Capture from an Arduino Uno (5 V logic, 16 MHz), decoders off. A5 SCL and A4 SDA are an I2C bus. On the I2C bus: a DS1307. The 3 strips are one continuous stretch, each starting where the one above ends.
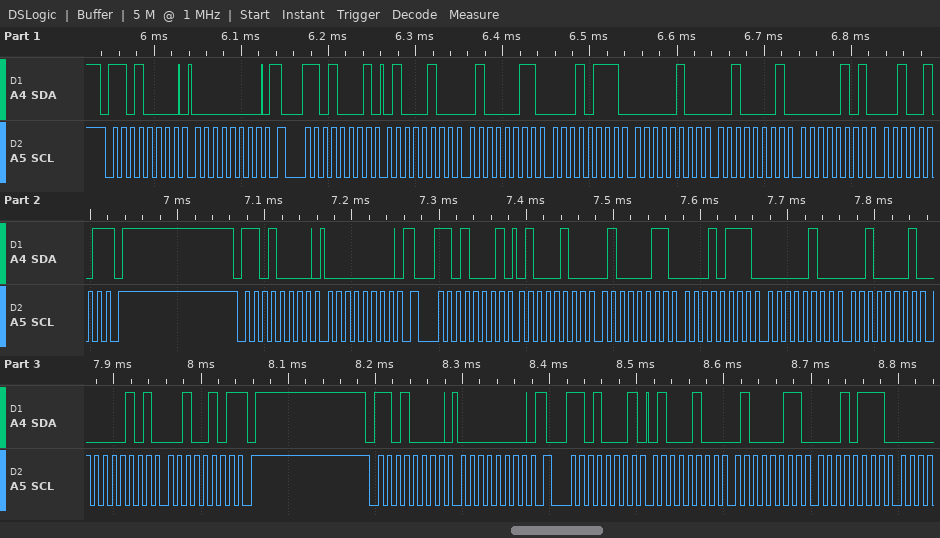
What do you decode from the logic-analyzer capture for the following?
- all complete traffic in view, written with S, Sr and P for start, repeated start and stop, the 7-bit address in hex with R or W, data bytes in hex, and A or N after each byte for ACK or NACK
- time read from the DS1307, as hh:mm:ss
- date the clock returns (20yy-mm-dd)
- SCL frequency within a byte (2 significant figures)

S 68W A 00 A Sr 68R A 44 A 43 A 17 A 04 A 21 A 05 A 25 N P S 68W A 00 A Sr 68R A 44 A 43 A 17 A 04 A 21 A 05 A 25 N P S 68W A 00 A Sr 68R A 44 A 43 A 17 A
17:43:44
2025-05-21
100 kHz
